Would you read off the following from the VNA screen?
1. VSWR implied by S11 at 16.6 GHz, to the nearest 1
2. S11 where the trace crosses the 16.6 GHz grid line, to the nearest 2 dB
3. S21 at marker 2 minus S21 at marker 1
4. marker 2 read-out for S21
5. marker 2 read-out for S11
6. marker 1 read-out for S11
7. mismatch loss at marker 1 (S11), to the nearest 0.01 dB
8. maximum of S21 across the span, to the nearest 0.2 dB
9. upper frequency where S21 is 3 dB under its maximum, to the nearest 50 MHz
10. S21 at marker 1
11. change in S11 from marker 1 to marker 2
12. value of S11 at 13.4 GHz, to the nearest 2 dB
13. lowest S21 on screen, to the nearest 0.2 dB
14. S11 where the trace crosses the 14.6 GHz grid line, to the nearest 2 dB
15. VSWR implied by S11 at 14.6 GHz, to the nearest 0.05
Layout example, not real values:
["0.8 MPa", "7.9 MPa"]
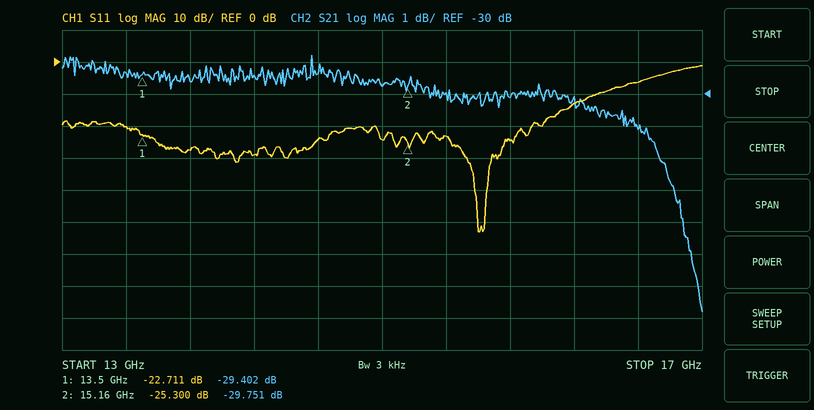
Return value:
["3", "-6 dB", "-0.349 dB", "-29.751 dB", "-25.300 dB", "-22.711 dB", "0.02 dB", "-28.8 dB", "16.70 GHz", "-29.402 dB", "-2.589 dB", "-20 dB", "-36.8 dB", "-24 dB", "1.15"]
